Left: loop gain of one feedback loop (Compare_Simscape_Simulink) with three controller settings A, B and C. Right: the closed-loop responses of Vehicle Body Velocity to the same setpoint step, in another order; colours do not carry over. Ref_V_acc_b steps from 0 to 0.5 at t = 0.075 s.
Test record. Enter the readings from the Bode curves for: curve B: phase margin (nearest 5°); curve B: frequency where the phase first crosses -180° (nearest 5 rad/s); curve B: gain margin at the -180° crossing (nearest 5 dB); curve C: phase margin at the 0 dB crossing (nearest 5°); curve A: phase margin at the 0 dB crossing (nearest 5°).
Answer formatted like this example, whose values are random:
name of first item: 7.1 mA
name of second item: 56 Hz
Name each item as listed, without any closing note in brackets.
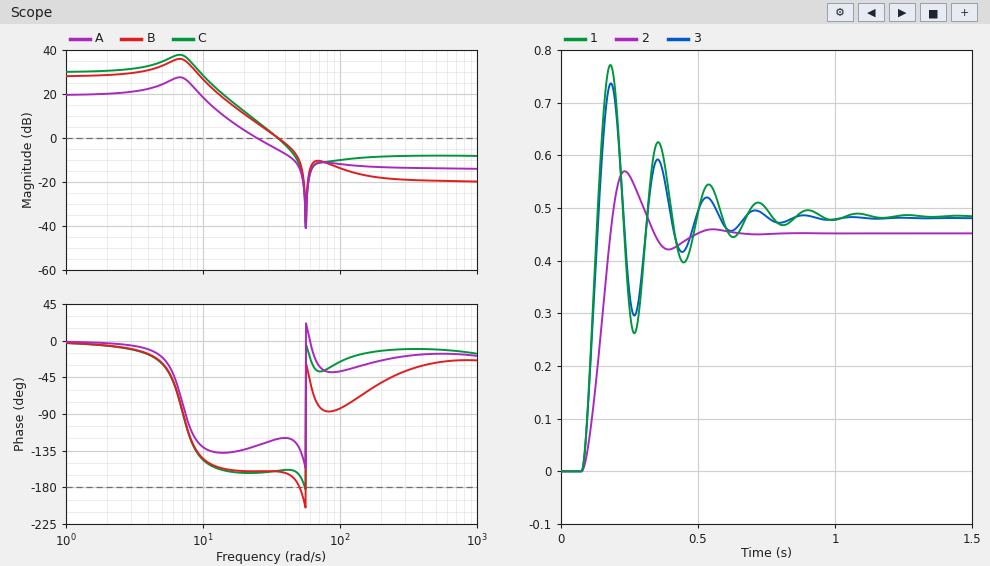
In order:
curve B: phase margin: 20°
curve B: frequency where the phase first crosses -180°: 50 rad/s
curve B: gain margin at the -180° crossing: 10 dB
curve C: phase margin at the 0 dB crossing: 20°
curve A: phase margin at the 0 dB crossing: 50°
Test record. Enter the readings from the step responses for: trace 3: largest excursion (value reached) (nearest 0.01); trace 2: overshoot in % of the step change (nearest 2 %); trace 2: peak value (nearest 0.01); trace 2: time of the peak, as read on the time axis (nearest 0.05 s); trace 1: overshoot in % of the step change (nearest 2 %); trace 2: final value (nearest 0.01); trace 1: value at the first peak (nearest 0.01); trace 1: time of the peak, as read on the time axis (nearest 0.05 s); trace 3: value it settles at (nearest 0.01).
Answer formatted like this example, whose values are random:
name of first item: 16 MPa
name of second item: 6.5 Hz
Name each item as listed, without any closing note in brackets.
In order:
trace 3: largest excursion (value reached): 0.74
trace 2: overshoot in % of the step change: 26 %
trace 2: peak value: 0.57
trace 2: time of the peak, as read on the time axis: 0.25 s
trace 1: overshoot in % of the step change: 60 %
trace 2: final value: 0.45
trace 1: value at the first peak: 0.77
trace 1: time of the peak, as read on the time axis: 0.20 s
trace 3: value it settles at: 0.48
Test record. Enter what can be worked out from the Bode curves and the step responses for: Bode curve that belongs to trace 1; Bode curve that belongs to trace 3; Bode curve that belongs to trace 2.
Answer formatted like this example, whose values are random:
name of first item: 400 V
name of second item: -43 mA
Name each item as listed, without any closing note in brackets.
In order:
Bode curve that belongs to trace 1: C
Bode curve that belongs to trace 3: B
Bode curve that belongs to trace 2: A
